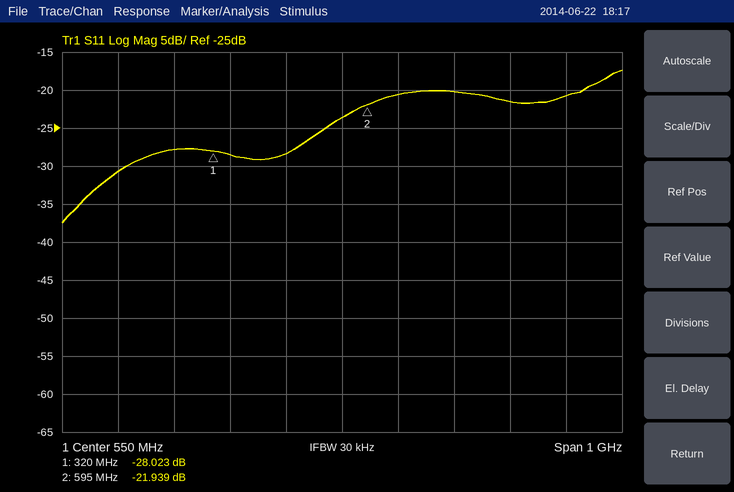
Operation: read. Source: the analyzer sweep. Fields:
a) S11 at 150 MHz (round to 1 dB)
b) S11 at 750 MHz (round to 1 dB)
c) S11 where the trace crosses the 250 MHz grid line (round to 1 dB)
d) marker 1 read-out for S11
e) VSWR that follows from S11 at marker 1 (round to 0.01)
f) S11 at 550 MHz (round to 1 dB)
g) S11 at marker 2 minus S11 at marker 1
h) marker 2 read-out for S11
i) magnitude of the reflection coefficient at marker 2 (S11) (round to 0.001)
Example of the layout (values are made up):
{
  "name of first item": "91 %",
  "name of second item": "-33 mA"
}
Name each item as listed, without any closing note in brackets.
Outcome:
{
  "S11 at 150 MHz": "-31 dB",
  "S11 at 750 MHz": "-20 dB",
  "S11 where the trace crosses the 250 MHz grid line": "-28 dB",
  "marker 1 read-out for S11": "-28.023 dB",
  "VSWR that follows from S11 at marker 1": "1.08",
  "S11 at 550 MHz": "-24 dB",
  "S11 at marker 2 minus S11 at marker 1": "6.084 dB",
  "marker 2 read-out for S11": "-21.939 dB",
  "magnitude of the reflection coefficient at marker 2 (S11)": "0.080"
}
